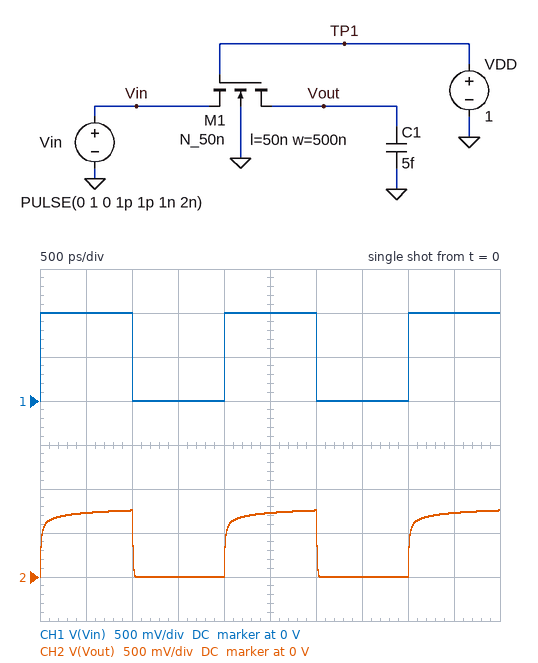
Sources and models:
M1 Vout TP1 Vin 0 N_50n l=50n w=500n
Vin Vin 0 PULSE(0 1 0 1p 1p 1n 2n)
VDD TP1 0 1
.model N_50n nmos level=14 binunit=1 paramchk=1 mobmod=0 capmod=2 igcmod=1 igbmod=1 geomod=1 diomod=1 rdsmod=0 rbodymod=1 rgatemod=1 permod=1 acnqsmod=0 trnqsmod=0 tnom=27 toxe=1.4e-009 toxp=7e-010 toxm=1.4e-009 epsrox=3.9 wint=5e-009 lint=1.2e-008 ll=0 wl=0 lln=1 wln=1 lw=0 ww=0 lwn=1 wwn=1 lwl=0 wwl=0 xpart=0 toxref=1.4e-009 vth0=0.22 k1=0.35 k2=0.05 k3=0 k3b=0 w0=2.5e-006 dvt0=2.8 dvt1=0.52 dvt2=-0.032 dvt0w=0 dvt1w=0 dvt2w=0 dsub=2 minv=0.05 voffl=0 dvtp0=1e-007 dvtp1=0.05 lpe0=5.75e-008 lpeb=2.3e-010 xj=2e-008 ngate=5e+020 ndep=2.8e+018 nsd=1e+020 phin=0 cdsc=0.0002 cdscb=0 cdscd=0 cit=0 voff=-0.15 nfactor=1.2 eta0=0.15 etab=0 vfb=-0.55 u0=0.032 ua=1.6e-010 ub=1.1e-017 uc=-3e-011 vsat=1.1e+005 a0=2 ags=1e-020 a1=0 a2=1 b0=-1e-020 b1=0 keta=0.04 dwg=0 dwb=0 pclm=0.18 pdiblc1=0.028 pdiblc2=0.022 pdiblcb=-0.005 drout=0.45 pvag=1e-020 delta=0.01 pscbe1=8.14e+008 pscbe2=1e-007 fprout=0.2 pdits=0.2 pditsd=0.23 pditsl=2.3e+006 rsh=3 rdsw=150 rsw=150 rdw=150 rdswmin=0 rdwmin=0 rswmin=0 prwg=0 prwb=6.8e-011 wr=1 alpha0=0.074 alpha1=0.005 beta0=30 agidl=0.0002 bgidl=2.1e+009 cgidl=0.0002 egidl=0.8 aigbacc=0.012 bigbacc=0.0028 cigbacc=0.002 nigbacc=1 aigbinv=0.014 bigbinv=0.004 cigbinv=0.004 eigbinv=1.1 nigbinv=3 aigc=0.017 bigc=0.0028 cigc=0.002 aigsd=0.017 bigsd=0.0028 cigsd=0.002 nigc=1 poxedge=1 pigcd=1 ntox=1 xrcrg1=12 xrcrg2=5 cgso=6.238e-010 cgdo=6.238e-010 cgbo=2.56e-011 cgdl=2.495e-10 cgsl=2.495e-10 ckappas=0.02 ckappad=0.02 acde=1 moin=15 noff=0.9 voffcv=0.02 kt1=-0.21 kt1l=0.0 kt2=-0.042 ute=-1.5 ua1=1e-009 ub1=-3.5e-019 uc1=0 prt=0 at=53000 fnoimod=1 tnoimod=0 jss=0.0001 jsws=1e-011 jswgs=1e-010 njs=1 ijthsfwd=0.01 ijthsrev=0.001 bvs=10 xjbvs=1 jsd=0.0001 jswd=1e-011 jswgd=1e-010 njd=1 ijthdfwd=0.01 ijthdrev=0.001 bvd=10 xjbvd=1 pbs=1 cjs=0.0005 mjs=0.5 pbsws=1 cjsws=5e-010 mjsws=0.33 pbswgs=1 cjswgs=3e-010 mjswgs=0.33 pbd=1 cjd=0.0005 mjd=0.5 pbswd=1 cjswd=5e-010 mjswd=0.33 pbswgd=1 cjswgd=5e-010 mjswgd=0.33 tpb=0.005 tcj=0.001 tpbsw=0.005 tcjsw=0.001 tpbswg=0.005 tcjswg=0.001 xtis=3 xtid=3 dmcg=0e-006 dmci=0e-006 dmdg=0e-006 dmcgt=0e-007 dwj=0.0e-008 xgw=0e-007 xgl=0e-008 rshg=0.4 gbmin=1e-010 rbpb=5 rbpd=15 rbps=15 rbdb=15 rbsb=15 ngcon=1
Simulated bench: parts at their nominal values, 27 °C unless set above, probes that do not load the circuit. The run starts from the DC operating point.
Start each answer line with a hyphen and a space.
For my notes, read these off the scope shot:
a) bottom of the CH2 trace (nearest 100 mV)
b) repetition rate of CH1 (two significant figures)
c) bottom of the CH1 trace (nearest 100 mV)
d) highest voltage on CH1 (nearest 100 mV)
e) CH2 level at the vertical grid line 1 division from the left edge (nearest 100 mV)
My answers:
- 0 V
- 500 MHz
- 0 V
- 1.0 V
- 700 mV
